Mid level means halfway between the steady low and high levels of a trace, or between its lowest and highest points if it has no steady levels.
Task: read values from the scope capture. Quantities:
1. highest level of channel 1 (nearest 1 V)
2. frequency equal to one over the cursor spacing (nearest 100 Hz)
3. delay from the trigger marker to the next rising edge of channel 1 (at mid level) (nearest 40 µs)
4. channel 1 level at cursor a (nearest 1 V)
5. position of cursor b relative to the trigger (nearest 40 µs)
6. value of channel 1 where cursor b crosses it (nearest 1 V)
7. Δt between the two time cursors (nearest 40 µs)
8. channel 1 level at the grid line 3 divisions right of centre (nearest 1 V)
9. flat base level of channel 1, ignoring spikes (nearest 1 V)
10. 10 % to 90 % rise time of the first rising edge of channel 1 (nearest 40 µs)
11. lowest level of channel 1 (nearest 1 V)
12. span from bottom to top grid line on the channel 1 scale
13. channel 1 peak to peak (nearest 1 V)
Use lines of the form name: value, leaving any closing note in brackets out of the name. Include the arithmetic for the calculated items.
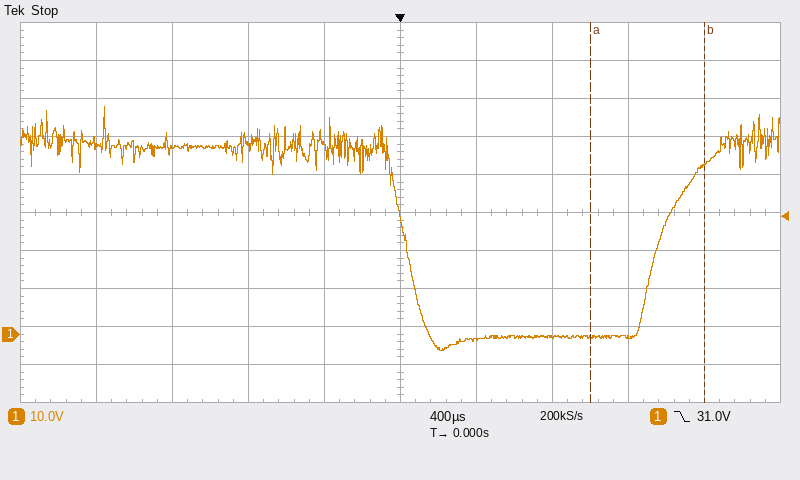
highest level of channel 1: 60 V
frequency equal to one over the cursor spacing: 1 / 600 µs ≈ 1.7 kHz
delay from the trigger marker to the next rising edge of channel 1 (at mid level): 1.36 ms
channel 1 level at cursor a: -1 V
position of cursor b relative to the trigger: +1.60 ms
value of channel 1 where cursor b crosses it: 45 V
Δt between the two time cursors: 600 µs
channel 1 level at the grid line 3 divisions right of centre: -1 V
flat base level of channel 1, ignoring spikes: -1 V
10 % to 90 % rise time of the first rising edge of channel 1: 320 µs
lowest level of channel 1: -4 V
span from bottom to top grid line on the channel 1 scale: 100 V
channel 1 peak to peak: 60 V − (-4 V) = 64 V
